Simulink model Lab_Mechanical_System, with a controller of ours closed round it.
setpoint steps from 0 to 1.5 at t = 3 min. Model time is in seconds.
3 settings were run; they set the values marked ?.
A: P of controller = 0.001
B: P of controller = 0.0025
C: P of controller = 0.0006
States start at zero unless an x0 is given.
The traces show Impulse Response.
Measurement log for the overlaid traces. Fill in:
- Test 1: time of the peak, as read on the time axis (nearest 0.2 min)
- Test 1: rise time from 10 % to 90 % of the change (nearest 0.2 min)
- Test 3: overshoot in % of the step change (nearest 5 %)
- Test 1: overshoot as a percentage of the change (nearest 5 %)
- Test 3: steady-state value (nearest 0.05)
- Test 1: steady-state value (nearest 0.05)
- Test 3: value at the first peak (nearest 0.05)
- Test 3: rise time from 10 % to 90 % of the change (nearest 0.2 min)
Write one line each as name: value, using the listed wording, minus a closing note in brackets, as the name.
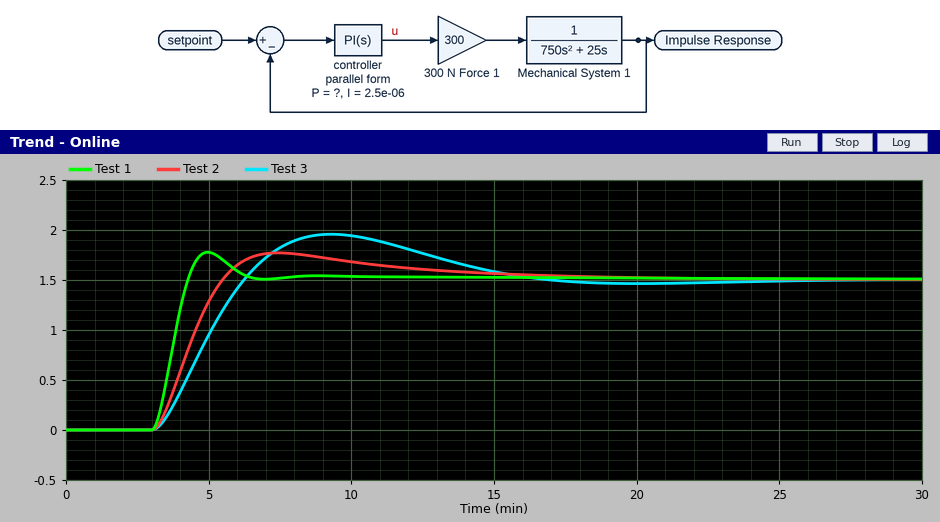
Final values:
Test 1: time of the peak, as read on the time axis: 5.0 min
Test 1: rise time from 10 % to 90 % of the change: 0.8 min
Test 3: overshoot in % of the step change: 30 %
Test 1: overshoot as a percentage of the change: 20 %
Test 3: steady-state value: 1.50
Test 1: steady-state value: 1.50
Test 3: value at the first peak: 1.95
Test 3: rise time from 10 % to 90 % of the change: 2.2 min
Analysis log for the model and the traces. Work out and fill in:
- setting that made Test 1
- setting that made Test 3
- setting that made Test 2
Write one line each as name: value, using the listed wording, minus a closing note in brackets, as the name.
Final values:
setting that made Test 1: B
setting that made Test 3: C
setting that made Test 2: A
